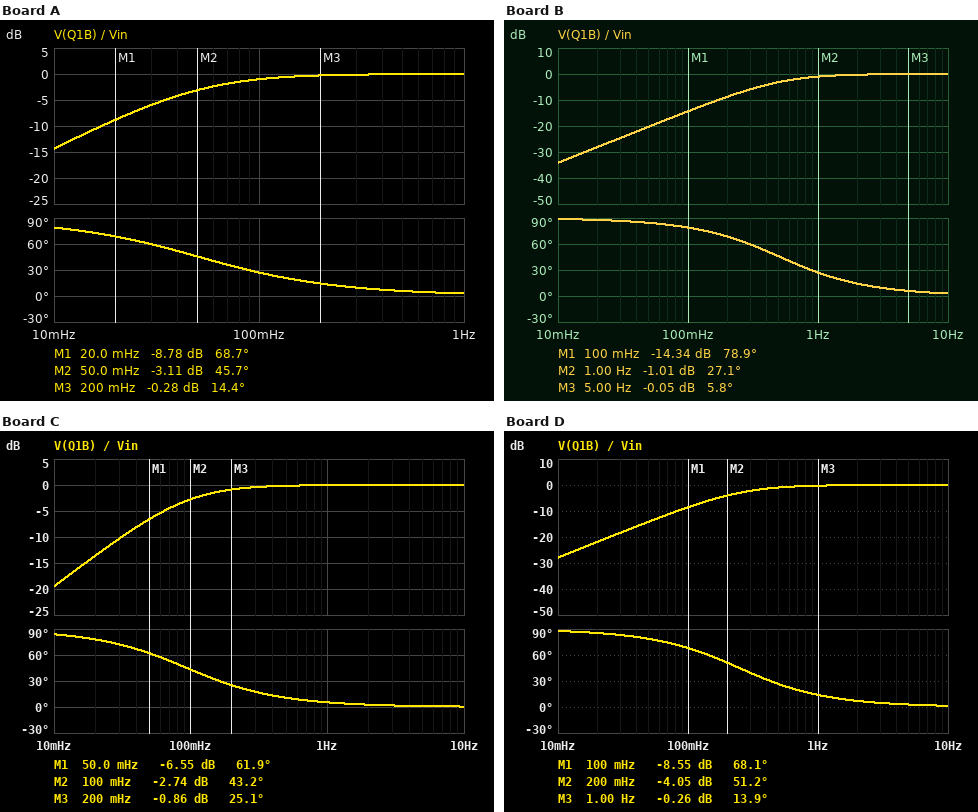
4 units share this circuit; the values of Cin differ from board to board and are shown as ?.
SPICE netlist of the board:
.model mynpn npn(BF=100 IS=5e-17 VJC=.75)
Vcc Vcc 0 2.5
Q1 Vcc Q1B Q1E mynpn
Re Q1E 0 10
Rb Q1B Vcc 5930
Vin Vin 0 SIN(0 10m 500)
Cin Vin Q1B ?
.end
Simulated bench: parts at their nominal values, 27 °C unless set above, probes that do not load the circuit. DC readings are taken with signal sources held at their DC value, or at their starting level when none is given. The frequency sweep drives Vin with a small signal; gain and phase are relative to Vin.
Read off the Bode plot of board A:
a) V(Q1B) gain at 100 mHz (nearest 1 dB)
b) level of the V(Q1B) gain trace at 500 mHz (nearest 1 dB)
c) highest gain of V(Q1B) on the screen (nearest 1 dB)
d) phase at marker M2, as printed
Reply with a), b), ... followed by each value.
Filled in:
a) -1 dB
b) 0 dB
c) 0 dB
d) 45.7 deg
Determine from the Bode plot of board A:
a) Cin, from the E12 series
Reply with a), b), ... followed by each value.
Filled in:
a) 3.3 mF
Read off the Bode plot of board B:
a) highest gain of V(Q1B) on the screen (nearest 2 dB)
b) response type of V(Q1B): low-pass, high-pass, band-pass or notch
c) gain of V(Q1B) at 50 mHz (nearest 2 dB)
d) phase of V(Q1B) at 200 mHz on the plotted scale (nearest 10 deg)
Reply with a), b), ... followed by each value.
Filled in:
a) 0 dB
b) high-pass
c) -20 dB
d) 70 deg
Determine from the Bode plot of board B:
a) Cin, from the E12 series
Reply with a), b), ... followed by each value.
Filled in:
a) 330 µF
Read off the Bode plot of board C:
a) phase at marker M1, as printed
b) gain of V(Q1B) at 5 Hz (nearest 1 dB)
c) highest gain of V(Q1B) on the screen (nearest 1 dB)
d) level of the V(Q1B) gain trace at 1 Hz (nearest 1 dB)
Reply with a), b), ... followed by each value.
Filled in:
a) 61.9 deg
b) 0 dB
c) 0 dB
d) 0 dB
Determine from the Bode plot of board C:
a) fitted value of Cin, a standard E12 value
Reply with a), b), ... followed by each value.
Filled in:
a) 1.8 mF
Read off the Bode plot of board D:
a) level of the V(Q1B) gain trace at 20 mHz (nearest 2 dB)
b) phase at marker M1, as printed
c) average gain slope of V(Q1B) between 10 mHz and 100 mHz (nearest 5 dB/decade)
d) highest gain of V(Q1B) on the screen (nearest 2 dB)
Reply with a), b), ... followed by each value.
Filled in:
a) -22 dB
b) 68.1 deg
c) 20 dB/decade
d) 0 dB
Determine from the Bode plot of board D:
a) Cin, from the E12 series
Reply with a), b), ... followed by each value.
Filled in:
a) 680 µF
